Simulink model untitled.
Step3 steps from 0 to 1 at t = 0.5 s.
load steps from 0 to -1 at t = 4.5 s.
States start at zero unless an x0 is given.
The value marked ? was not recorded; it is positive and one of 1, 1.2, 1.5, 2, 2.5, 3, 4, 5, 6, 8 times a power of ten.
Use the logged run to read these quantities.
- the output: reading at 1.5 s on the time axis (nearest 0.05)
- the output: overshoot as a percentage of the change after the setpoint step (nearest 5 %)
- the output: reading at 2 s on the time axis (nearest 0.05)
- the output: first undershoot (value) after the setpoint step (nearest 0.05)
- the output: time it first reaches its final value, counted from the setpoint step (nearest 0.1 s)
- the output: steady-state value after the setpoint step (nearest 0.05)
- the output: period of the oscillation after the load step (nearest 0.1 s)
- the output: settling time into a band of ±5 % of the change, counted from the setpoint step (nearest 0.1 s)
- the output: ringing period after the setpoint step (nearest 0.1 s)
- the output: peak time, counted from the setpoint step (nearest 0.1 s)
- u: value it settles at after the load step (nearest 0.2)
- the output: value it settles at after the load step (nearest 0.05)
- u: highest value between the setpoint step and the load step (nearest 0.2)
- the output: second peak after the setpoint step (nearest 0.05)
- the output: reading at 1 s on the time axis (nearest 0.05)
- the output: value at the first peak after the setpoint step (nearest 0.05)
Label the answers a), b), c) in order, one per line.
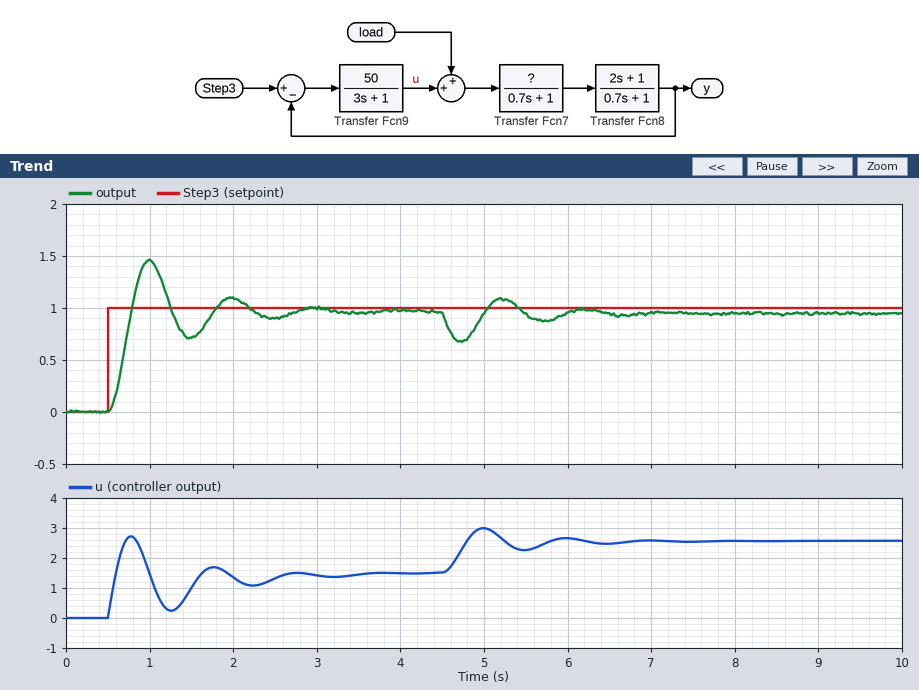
a) 0.70
b) 50 %
c) 1.10
d) 0.70
e) 0.3 s
f) 0.95
g) 1.0 s
h) 2.1 s
i) 1.0 s
j) 0.5 s
k) 2.6
l) 0.95
m) 2.8
n) 1.10
o) 1.45
p) 1.45
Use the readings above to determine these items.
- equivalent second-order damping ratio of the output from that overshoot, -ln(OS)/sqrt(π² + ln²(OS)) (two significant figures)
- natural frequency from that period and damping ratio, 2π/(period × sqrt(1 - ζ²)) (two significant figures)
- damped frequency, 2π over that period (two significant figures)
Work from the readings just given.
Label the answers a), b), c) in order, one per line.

a) 0.22
b) 6.4 rad/s
c) 6.3 rad/s
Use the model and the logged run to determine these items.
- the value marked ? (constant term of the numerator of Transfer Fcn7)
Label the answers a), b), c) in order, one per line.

a) 0.6
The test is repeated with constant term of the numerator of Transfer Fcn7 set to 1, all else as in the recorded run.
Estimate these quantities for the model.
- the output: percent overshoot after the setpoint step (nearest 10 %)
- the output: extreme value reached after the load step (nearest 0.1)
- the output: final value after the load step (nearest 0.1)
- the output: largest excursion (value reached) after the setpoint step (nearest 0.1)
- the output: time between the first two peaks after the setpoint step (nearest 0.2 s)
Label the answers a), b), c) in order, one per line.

a) 60 %
b) 0.6
c) 1.0
d) 1.6
e) 0.8 s
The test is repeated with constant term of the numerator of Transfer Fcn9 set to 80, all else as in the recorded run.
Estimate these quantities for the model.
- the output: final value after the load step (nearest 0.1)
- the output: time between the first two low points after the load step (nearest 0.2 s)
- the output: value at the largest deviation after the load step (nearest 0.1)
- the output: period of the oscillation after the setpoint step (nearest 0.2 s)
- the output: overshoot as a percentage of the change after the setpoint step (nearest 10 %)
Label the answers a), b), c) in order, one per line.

a) 1.0
b) 0.8 s
c) 0.7
d) 0.8 s
e) 60 %
